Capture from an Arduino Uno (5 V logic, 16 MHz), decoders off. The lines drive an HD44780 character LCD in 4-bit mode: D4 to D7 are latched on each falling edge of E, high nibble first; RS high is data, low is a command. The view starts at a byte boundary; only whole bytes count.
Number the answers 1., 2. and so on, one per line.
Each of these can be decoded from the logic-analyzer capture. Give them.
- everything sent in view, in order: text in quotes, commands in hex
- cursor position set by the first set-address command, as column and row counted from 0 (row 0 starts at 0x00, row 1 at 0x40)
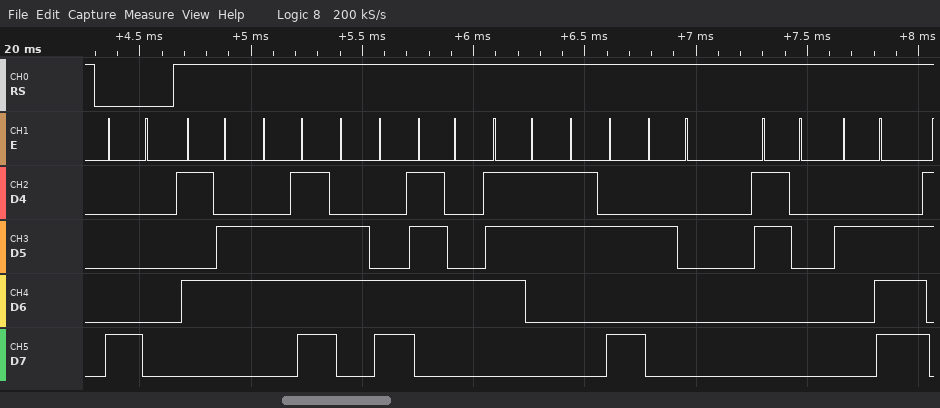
1. 0x80 "Volts: 0."
2. column 0, row 0
